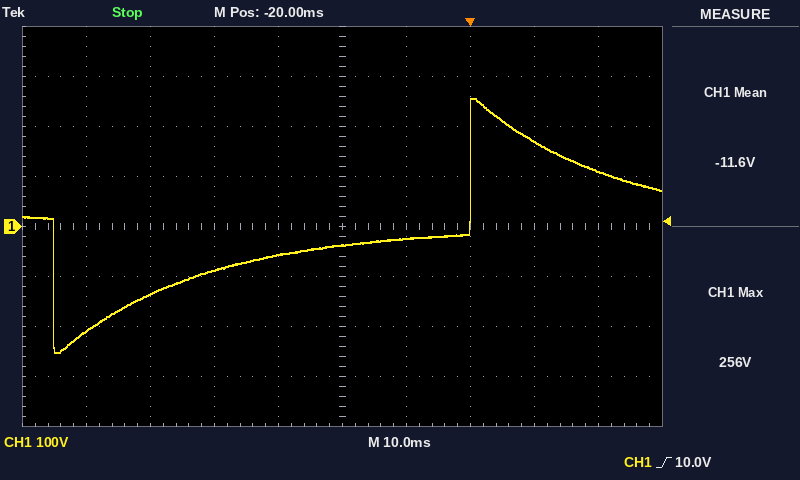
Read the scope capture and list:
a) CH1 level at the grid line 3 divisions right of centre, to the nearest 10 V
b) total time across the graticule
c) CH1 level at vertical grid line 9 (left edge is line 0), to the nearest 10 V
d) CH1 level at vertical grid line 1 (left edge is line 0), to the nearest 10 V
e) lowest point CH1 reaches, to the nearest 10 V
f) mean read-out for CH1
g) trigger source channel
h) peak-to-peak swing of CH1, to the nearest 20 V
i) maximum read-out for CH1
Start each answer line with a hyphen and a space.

- 170 V
- 100 ms
- 110 V
- -210 V
- -250 V
- -11.6 V
- CH1
- 500 V
- 256 V
